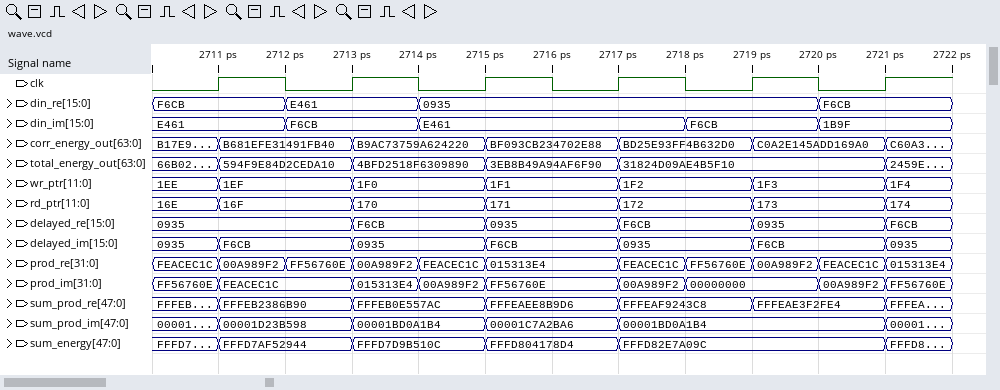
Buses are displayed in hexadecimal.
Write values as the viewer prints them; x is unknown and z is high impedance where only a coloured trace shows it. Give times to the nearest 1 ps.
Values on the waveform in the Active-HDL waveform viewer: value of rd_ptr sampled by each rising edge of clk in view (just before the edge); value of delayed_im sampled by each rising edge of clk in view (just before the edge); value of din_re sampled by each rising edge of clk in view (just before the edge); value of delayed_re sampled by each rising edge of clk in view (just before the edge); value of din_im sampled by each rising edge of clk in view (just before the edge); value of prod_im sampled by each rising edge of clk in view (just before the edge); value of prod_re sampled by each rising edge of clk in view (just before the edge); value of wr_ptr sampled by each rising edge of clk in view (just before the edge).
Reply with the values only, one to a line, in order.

16E, 16F, 170, 171, 172, 173
0935, F6CB, 0935, F6CB, 0935, F6CB
F6CB, E461, 0935, 0935, 0935, F6CB
0935, 0935, F6CB, 0935, F6CB, 0935
E461, F6CB, E461, E461, F6CB, 1B9F
FF56760E, FEACEC1C, 00A989F2, FF56760E, 00000000, 00A989F2
FEACEC1C, FF56760E, FEACEC1C, 015313E4, FF56760E, FEACEC1C
1EE, 1EF, 1F0, 1F1, 1F2, 1F3
